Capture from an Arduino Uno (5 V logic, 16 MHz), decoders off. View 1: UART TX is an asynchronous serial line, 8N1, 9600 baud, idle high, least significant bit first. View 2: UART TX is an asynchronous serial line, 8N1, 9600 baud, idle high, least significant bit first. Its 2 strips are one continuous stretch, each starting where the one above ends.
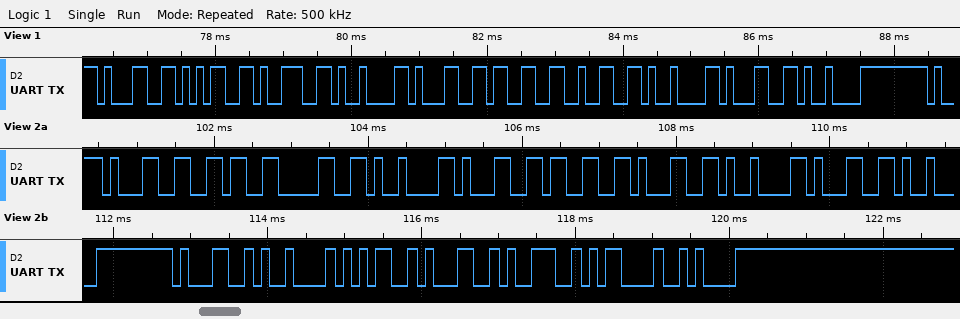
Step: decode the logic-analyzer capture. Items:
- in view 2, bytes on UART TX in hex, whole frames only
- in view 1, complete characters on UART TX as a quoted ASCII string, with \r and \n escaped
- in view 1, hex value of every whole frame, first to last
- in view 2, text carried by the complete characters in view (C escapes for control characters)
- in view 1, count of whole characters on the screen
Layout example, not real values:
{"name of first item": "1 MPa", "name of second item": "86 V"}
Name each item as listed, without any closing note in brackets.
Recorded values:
{"in view 2, bytes on UART TX in hex, whole frames only": "31 36 30 09 31 33 31 09 31 09 31 09 35 31 39 0D 0A", "in view 1, complete characters on UART TX as a quoted ASCII string, with \\r and \\n escaped": "\"159\\t132\\t1\\t\"", "in view 1, hex value of every whole frame, first to last": "31 35 39 09 31 33 32 09 31 09", "in view 2, text carried by the complete characters in view": "\"160\\t131\\t1\\t1\\t519\\r\\n\"", "in view 1, count of whole characters on the screen": "10"}
